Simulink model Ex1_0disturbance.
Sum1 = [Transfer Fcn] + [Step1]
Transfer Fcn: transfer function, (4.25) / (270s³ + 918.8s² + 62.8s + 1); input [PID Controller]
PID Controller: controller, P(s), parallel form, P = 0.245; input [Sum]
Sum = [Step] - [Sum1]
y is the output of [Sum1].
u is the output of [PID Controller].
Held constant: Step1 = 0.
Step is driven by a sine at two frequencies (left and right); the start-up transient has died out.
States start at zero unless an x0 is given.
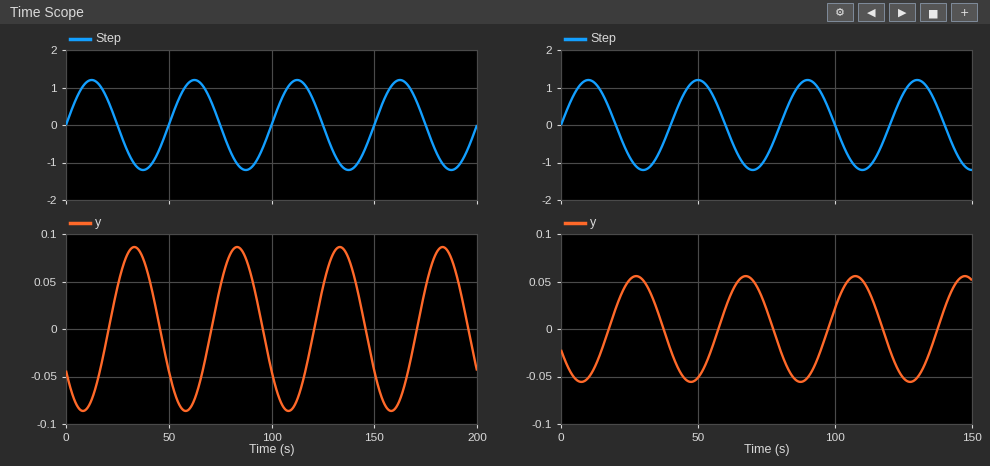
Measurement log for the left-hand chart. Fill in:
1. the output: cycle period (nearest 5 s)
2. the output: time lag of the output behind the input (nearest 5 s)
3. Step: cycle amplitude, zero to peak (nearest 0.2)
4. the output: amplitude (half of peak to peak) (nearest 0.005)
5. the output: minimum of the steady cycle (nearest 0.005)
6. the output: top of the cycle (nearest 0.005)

50 s
20 s
1.2
0.085
-0.085
0.085
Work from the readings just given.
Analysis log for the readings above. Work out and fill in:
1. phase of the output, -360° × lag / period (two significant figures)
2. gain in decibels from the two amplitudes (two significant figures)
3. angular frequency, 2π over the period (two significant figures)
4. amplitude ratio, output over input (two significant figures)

-140°
-23 dB
0.13 rad/s
0.071
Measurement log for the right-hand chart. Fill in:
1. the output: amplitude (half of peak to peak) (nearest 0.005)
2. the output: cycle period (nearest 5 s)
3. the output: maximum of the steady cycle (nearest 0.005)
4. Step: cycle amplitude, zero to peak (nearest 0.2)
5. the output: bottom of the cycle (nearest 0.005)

0.055
40 s
0.055
1.2
-0.055
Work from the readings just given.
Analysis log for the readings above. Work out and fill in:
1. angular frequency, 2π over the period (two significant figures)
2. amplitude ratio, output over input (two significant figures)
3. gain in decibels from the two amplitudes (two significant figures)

0.16 rad/s
0.046
-27 dB
